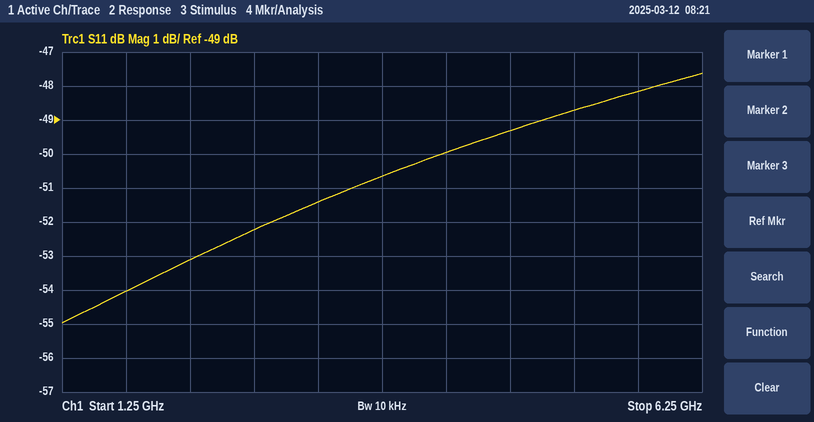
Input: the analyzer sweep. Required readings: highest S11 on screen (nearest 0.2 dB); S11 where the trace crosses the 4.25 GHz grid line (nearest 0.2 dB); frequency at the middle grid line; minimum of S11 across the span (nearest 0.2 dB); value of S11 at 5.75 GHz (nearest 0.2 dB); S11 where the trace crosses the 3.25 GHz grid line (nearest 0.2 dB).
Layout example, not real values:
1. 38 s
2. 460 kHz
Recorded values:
1. -47.6 dB
2. -50.0 dB
3. 3.75 GHz
4. -55.0 dB
5. -48.2 dB
6. -51.4 dB
